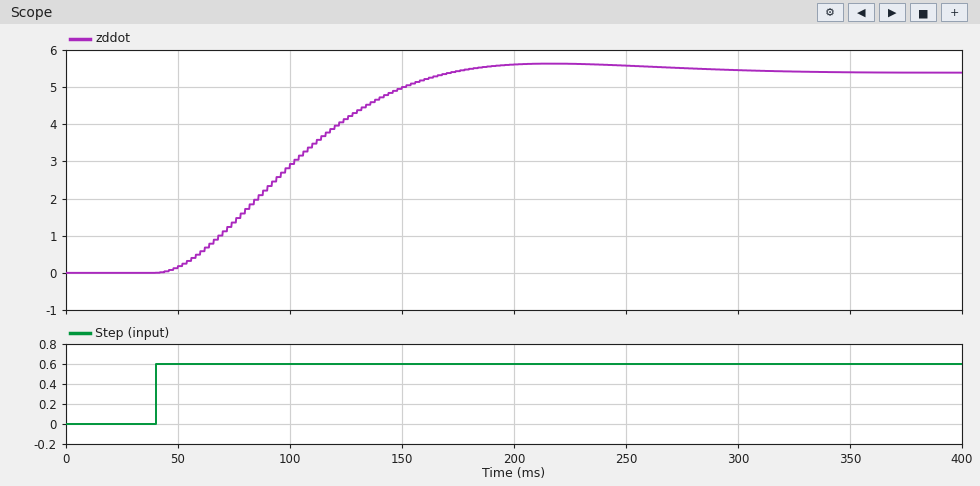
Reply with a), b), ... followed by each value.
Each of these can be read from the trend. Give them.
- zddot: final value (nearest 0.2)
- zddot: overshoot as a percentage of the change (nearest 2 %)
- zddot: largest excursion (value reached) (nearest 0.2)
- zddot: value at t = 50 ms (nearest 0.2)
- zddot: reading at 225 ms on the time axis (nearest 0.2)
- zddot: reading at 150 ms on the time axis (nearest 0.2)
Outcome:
a) 5.4
b) 4 %
c) 5.6
d) 0.2
e) 5.6
f) 5.0
